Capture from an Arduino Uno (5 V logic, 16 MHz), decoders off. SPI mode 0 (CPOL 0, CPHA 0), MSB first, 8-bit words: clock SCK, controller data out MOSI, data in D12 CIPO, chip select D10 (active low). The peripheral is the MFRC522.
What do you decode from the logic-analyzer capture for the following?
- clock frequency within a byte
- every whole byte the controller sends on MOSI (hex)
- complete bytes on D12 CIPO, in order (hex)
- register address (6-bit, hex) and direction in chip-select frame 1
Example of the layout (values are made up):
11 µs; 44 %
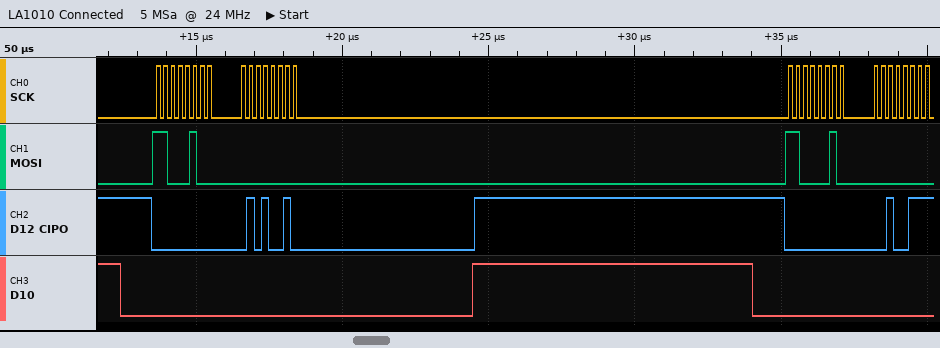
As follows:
4 MHz; C4 00 C2 00; 00 52 00 27; 0x22 read
